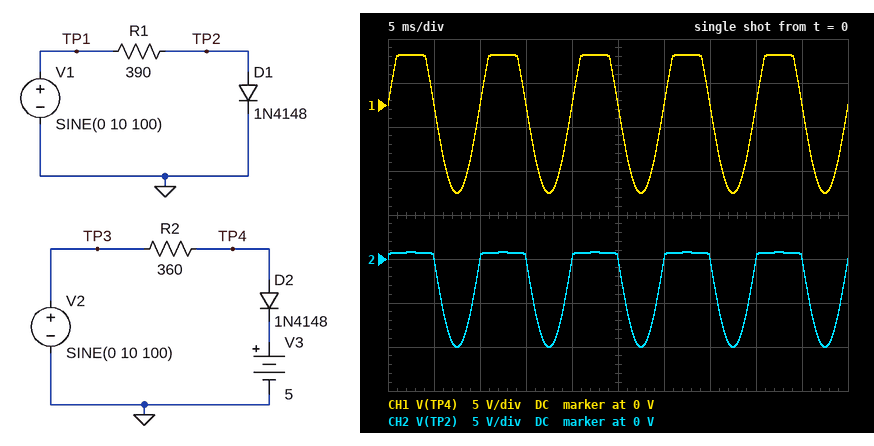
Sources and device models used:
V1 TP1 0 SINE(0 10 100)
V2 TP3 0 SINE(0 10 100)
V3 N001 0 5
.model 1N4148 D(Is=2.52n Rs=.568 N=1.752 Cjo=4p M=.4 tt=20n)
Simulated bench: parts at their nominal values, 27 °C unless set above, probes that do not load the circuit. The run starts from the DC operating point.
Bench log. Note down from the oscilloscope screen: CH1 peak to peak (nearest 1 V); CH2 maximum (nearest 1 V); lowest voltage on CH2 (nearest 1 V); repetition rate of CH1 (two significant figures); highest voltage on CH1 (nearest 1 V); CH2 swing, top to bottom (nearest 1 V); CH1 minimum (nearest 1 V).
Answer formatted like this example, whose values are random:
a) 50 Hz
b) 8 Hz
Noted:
a) 16 V
b) 1 V
c) -10 V
d) 100 Hz
e) 6 V
f) 11 V
g) -10 V
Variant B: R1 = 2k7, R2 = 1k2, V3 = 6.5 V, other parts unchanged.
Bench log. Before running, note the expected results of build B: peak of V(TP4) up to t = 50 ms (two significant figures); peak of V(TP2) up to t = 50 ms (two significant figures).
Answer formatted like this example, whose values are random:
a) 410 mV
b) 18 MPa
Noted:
a) 7.1 V
b) 640 mV
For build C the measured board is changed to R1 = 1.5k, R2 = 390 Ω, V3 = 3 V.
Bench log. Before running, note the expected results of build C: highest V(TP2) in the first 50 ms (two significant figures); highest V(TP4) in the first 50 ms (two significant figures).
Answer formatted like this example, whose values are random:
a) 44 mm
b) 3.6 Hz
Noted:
a) 670 mV
b) 3.7 V
